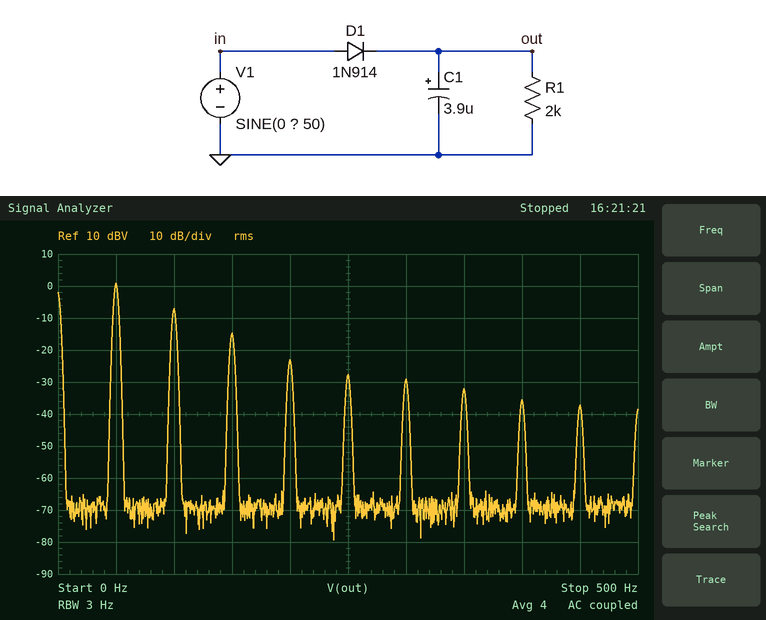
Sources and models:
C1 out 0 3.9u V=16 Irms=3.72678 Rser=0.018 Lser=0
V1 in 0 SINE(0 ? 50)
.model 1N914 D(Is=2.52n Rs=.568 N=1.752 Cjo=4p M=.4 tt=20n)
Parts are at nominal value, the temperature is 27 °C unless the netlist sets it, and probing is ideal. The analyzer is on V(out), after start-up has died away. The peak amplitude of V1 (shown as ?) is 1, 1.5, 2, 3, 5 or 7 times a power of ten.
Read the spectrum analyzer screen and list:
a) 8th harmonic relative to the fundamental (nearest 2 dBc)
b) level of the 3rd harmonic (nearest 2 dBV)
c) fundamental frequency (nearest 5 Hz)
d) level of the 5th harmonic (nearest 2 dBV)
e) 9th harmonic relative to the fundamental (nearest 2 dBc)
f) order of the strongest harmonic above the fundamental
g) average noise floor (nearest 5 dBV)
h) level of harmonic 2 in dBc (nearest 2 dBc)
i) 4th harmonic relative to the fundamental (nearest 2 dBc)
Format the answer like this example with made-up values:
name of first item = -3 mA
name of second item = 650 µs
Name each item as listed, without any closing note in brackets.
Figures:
8th harmonic relative to the fundamental = -36 dBc
level of the 3rd harmonic = -14 dBV
fundamental frequency = 50 Hz
level of the 5th harmonic = -28 dBV
9th harmonic relative to the fundamental = -38 dBc
order of the strongest harmonic above the fundamental = 2
average noise floor = -70 dBV
level of harmonic 2 in dBc = -8 dBc
4th harmonic relative to the fundamental = -24 dBc
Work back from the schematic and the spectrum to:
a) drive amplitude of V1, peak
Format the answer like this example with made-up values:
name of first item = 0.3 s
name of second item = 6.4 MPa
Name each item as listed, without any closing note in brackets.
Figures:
drive amplitude of V1, peak = 5 V
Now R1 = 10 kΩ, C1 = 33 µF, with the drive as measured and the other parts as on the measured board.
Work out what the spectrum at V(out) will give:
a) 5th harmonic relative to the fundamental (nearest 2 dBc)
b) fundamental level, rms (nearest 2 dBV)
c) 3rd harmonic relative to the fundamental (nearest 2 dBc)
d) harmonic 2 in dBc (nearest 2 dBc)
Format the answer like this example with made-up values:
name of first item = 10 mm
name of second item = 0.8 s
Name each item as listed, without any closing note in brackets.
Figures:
5th harmonic relative to the fundamental = -16 dBc
fundamental level, rms = -24 dBV
3rd harmonic relative to the fundamental = -10 dBc
harmonic 2 in dBc = -6 dBc
